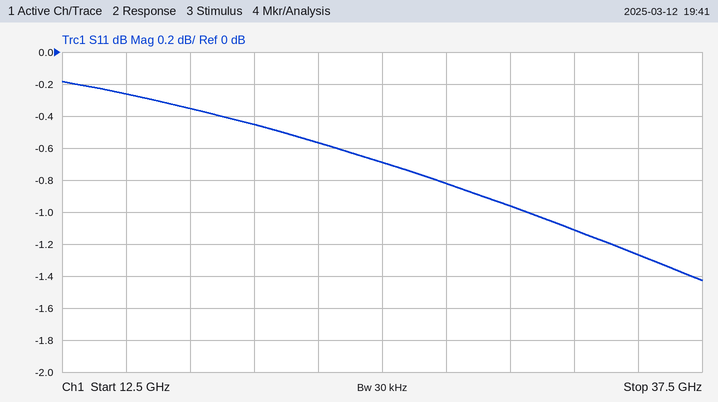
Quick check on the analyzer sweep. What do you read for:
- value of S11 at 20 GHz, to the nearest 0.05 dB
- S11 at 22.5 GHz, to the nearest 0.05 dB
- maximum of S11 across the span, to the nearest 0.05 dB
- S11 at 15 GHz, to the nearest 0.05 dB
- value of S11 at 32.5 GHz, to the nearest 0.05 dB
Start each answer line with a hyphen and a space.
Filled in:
- -0.45 dB
- -0.55 dB
- -0.20 dB
- -0.25 dB
- -1.10 dB
